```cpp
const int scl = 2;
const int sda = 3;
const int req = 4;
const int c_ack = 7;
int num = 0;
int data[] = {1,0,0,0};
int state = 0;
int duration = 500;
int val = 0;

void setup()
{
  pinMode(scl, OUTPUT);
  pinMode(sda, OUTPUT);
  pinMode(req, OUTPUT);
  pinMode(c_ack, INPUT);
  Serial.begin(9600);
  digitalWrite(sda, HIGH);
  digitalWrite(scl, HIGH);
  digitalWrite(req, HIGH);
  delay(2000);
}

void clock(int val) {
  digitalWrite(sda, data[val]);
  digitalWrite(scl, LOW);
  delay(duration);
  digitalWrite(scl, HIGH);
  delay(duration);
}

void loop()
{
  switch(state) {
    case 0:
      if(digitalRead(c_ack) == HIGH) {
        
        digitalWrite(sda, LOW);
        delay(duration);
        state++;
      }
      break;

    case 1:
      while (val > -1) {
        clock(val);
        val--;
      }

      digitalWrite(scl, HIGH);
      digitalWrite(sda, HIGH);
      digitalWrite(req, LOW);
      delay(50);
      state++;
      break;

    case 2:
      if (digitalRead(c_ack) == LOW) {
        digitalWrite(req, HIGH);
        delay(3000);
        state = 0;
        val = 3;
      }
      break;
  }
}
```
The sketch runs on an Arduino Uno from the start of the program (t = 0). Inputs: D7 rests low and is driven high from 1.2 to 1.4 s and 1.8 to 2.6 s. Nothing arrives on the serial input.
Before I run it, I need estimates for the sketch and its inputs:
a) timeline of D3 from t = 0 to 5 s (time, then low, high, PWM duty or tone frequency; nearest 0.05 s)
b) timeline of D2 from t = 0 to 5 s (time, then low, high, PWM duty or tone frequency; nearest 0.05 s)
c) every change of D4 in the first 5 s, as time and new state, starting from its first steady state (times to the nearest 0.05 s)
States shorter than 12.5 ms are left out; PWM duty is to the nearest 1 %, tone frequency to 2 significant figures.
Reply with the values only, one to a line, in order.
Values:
0 s high; 2 s low; 2.5 s high
0 s high; 2.5 s low; 3 s high
0 s high; 3.5 s low; 3.55 s high
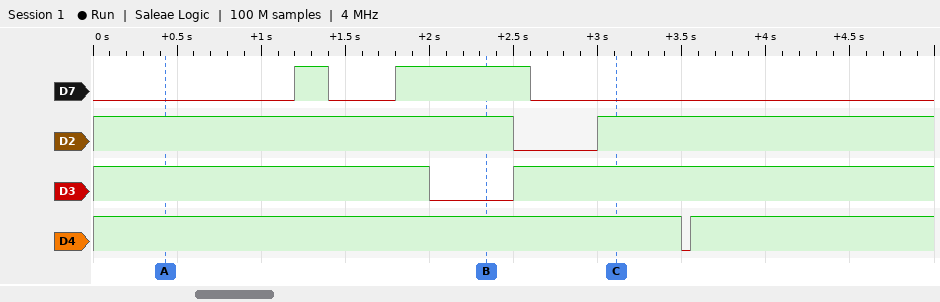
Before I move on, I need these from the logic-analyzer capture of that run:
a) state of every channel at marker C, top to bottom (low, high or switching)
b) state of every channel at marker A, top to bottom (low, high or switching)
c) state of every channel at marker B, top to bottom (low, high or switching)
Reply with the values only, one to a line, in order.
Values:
D7 low, D2 high, D3 high, D4 high
D7 low, D2 high, D3 high, D4 high
D7 high, D2 high, D3 low, D4 high
